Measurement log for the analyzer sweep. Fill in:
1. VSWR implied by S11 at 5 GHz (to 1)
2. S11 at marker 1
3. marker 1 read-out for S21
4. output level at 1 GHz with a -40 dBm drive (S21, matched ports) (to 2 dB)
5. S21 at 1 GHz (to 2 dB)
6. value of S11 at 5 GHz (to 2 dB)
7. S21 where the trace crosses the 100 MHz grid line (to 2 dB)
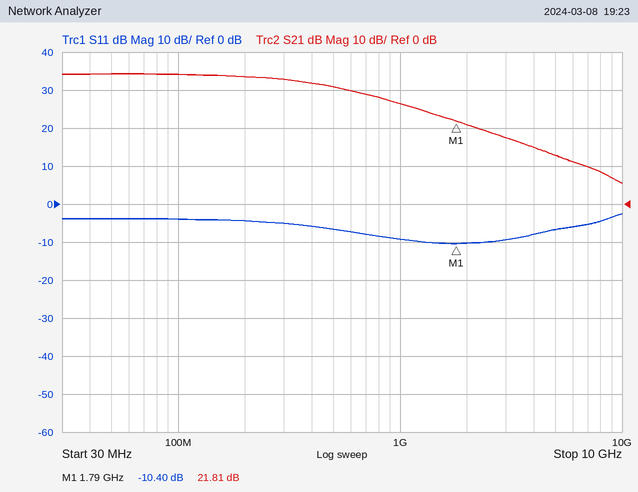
3
-10.40 dB
21.81 dB
-14 dBm
26 dB
-6 dB
34 dB
